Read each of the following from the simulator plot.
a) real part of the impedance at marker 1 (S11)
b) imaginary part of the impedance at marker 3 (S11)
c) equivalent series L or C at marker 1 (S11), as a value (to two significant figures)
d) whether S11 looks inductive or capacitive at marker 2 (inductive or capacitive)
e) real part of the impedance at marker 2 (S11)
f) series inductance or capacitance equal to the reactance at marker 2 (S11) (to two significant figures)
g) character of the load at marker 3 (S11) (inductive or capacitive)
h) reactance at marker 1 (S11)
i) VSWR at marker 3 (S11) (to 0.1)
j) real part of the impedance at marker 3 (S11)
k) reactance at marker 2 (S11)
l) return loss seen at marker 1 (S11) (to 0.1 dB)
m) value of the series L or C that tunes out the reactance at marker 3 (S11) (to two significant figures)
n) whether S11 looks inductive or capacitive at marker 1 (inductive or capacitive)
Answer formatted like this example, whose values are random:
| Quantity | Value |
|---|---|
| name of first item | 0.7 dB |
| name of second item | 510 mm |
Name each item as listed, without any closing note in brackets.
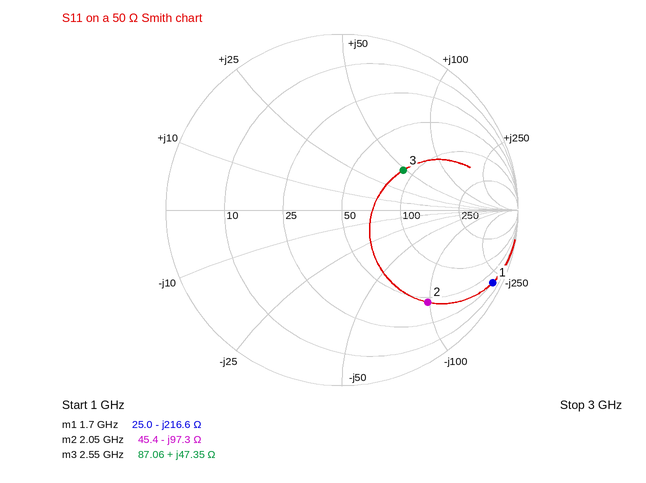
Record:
| Quantity | Value |
|---|---|
| real part of the impedance at marker 1 | 25.0 Ω |
| imaginary part of the impedance at marker 3 | +47.35 Ω |
| equivalent series L or C at marker 1 (S11), as a value | 430 fF |
| whether S11 looks inductive or capacitive at marker 2 | capacitive |
| real part of the impedance at marker 2 | 45.4 Ω |
| series inductance or capacitance equal to the reactance at marker 2 (S11) | 800 fF |
| character of the load at marker 3 (S11) | inductive |
| reactance at marker 1 | -216.6 Ω |
| VSWR at marker 3 (S11) | 2.4 |
| real part of the impedance at marker 3 | 87.06 Ω |
| reactance at marker 2 | -97.3 Ω |
| return loss seen at marker 1 (S11) | 0.4 dB |
| value of the series L or C that tunes out the reactance at marker 3 (S11) | 1.3 pF |
| whether S11 looks inductive or capacitive at marker 1 | capacitive |
